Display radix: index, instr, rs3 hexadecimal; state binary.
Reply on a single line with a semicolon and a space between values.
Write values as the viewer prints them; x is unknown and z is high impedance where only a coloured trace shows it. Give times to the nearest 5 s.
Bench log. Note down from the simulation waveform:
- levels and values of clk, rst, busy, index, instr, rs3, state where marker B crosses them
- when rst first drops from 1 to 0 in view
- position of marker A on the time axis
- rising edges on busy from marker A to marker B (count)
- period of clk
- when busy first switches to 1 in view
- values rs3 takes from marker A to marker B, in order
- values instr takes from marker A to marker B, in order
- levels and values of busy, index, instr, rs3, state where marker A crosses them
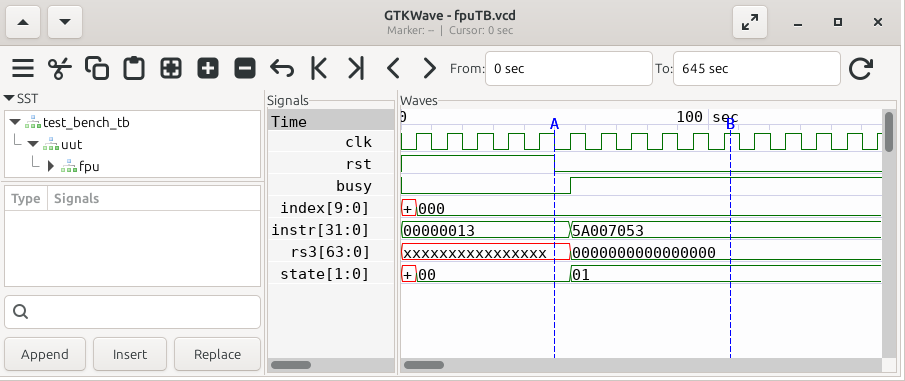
clk=1, rst=0, busy=1, index=000, instr=5A007053, rs3=0000000000000000, state=01; 50 s; 50 s; 1; 10 s; 55 s; xxxxxxxxxxxxxxxx, 0000000000000000; 00000013, 5A007053; busy=0, index=000, instr=00000013, rs3=xxxxxxxxxxxxxxxx, state=00
